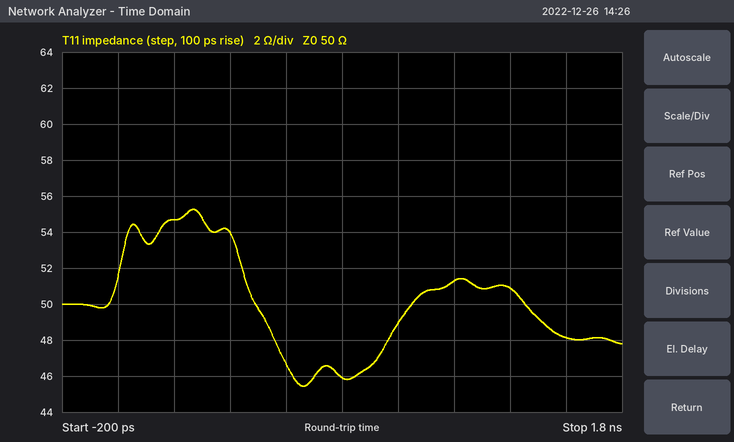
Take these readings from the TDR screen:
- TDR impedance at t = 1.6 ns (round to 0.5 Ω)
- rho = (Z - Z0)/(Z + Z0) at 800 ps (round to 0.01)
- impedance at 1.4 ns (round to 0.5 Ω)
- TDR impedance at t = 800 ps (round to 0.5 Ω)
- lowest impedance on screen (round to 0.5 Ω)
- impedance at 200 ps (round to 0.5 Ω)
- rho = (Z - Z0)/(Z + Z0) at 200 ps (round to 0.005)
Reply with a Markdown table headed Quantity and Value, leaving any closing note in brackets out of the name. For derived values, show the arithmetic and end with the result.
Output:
| Quantity | Value |
|---|---|
| TDR impedance at t = 1.6 ns | 48.0 Ω |
| rho = (Z - Z0)/(Z + Z0) at 800 ps | (46 − 50)/(46 + 50) ≈ -0.04 |
| impedance at 1.4 ns | 51.0 Ω |
| TDR impedance at t = 800 ps | 46.0 Ω |
| lowest impedance on screen | 45.5 Ω |
| impedance at 200 ps | 54.5 Ω |
| rho = (Z - Z0)/(Z + Z0) at 200 ps | (54.5 − 50)/(54.5 + 50) ≈ +0.0431, so +0.045 to the nearest 0.005 |
